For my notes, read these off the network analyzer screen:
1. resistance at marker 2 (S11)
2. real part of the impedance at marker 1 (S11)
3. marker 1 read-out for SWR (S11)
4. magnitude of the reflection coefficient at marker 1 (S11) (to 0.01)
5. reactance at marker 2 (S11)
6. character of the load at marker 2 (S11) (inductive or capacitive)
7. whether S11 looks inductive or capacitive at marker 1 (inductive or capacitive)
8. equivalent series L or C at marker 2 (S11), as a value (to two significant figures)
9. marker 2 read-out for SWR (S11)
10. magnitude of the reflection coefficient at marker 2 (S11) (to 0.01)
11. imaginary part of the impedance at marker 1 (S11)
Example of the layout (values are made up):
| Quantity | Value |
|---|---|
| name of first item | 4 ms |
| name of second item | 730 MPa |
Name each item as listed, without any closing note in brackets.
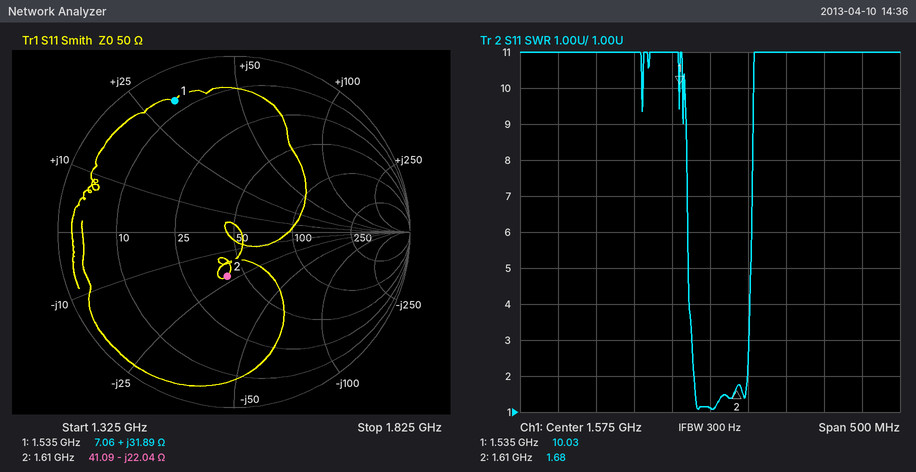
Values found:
| Quantity | Value |
|---|---|
| resistance at marker 2 | 41.09 Ω |
| real part of the impedance at marker 1 | 7.06 Ω |
| marker 1 read-out for SWR | 10.03 |
| magnitude of the reflection coefficient at marker 1 (S11) | 0.82 |
| reactance at marker 2 | -22.04 Ω |
| character of the load at marker 2 (S11) | capacitive |
| whether S11 looks inductive or capacitive at marker 1 | inductive |
| equivalent series L or C at marker 2 (S11), as a value | 4.5 pF |
| marker 2 read-out for SWR | 1.68 |
| magnitude of the reflection coefficient at marker 2 (S11) | 0.25 |
| imaginary part of the impedance at marker 1 | +31.89 Ω |
